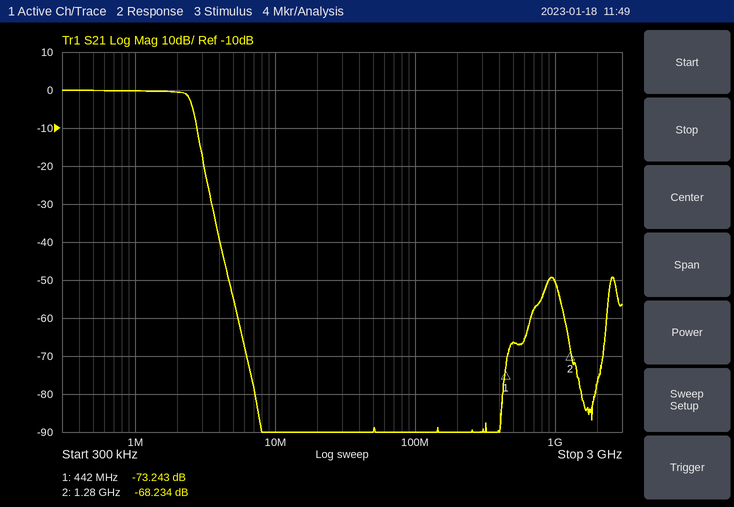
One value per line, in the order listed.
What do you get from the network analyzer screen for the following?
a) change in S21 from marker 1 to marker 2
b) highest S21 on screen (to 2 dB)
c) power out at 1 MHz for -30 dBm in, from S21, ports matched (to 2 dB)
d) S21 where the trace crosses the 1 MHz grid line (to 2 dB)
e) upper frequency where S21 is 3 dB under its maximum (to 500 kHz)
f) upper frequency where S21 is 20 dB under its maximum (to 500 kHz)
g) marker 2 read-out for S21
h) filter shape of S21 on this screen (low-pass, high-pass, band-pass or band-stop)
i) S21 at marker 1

5.009 dB
0 dB
-30 dBm
0 dB
2.5 MHz
3.0 MHz
-68.234 dB
low-pass
-73.243 dB
